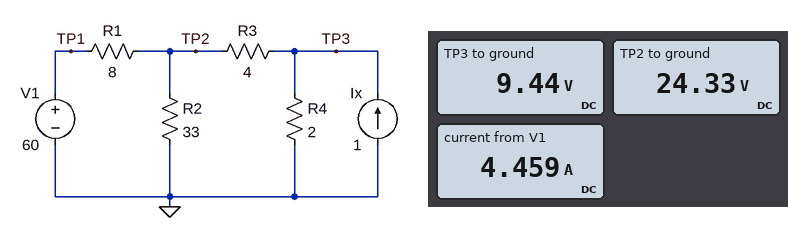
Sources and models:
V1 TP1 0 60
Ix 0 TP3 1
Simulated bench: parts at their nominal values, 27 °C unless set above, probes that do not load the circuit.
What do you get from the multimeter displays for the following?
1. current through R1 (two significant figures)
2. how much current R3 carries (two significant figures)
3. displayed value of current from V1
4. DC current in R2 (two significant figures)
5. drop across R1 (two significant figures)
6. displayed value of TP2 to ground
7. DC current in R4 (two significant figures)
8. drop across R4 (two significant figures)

4.5 A
3.7 A
4.459 A
740 mA
36 V
24.33 V
4.7 A
9.4 V
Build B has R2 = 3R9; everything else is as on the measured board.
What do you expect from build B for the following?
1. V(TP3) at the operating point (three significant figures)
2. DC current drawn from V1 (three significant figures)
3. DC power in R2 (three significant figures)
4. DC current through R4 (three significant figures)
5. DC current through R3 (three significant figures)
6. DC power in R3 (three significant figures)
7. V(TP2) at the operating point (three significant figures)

6.10 V
5.71 A
52.4 W
3.05 A
2.05 A
16.8 W
14.3 V
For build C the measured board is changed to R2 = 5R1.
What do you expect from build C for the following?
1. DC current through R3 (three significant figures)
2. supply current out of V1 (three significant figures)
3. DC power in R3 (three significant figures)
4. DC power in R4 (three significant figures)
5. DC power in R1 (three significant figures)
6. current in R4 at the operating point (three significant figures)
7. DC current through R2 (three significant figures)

2.34 A
5.49 A
22.0 W
22.4 W
241 W
3.34 A
3.15 A
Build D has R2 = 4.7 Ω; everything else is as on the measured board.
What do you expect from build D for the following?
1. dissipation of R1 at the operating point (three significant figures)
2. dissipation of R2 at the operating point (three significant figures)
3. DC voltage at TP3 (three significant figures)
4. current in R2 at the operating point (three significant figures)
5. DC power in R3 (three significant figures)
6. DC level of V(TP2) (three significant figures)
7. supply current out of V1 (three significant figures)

247 W
51.3 W
6.51 V
3.30 A
20.3 W
15.5 V
5.56 A
